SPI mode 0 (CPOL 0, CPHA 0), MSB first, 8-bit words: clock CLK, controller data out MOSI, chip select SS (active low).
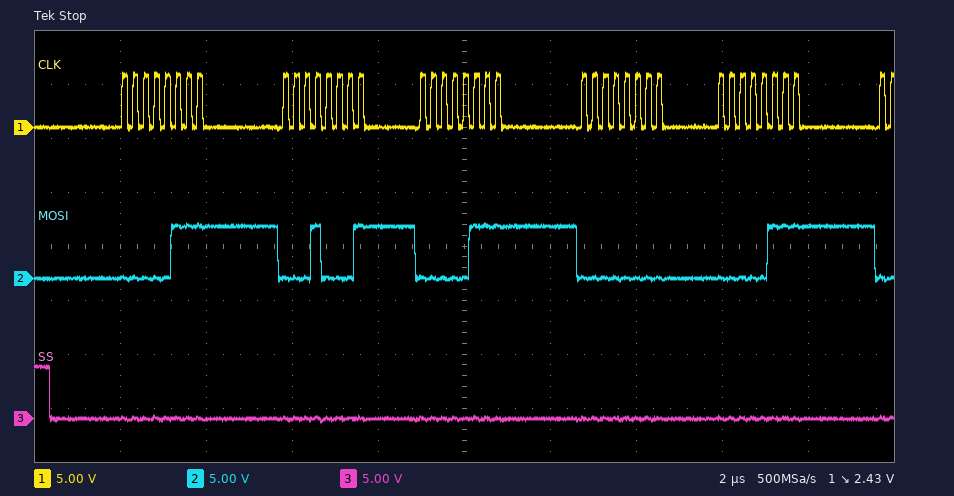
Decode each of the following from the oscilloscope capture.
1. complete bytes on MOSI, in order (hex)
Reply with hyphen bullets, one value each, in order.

- 07 11 07 00 07
